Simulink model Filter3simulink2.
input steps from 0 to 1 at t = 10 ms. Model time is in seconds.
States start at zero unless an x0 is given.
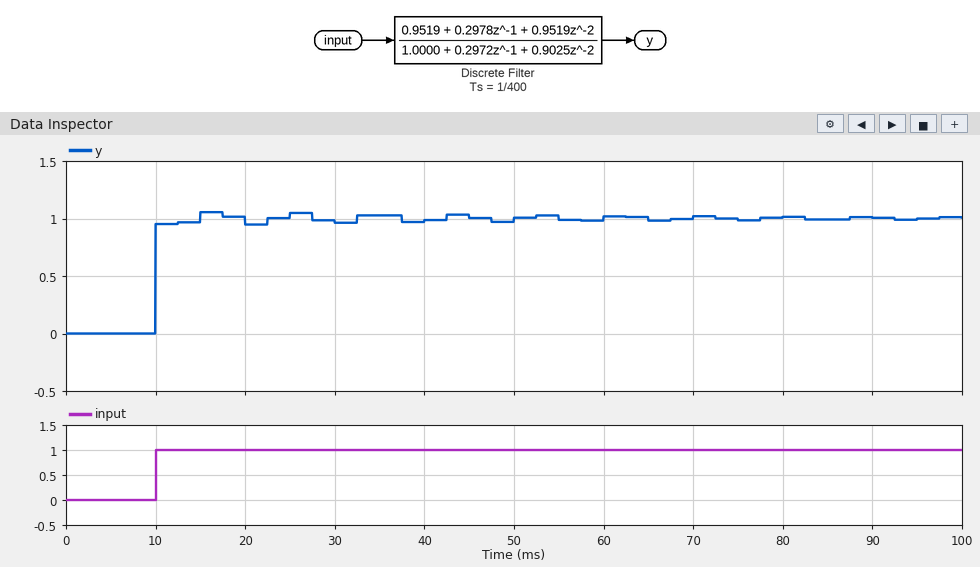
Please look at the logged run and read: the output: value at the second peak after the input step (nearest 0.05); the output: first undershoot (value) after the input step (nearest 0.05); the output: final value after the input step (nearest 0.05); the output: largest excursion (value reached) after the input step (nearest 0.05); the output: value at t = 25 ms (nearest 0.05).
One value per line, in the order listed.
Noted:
1.05
0.95
1.00
1.05
1.05
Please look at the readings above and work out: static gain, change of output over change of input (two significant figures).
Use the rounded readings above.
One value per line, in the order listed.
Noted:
1.0
